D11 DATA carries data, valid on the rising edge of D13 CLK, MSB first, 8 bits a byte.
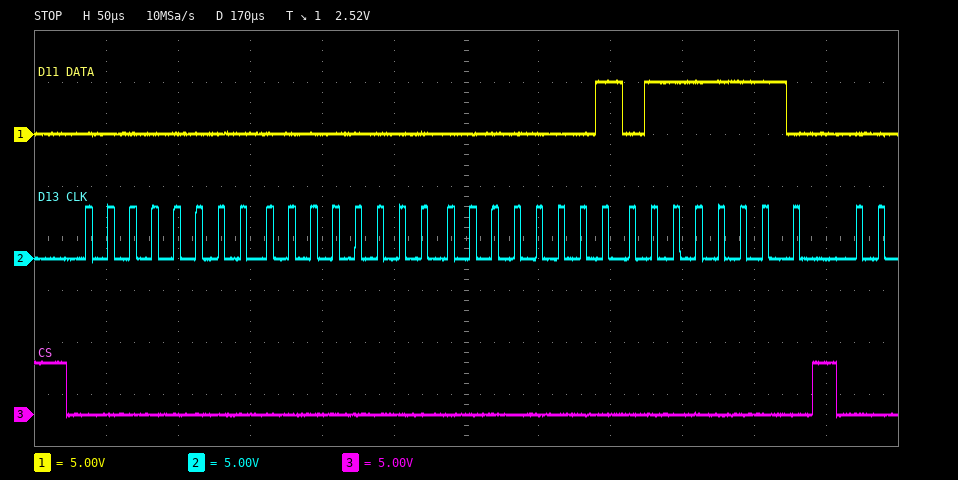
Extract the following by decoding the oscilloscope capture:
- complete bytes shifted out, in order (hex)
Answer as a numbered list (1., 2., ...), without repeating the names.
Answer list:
1. 0x00 0x00 0x01 0x7E
